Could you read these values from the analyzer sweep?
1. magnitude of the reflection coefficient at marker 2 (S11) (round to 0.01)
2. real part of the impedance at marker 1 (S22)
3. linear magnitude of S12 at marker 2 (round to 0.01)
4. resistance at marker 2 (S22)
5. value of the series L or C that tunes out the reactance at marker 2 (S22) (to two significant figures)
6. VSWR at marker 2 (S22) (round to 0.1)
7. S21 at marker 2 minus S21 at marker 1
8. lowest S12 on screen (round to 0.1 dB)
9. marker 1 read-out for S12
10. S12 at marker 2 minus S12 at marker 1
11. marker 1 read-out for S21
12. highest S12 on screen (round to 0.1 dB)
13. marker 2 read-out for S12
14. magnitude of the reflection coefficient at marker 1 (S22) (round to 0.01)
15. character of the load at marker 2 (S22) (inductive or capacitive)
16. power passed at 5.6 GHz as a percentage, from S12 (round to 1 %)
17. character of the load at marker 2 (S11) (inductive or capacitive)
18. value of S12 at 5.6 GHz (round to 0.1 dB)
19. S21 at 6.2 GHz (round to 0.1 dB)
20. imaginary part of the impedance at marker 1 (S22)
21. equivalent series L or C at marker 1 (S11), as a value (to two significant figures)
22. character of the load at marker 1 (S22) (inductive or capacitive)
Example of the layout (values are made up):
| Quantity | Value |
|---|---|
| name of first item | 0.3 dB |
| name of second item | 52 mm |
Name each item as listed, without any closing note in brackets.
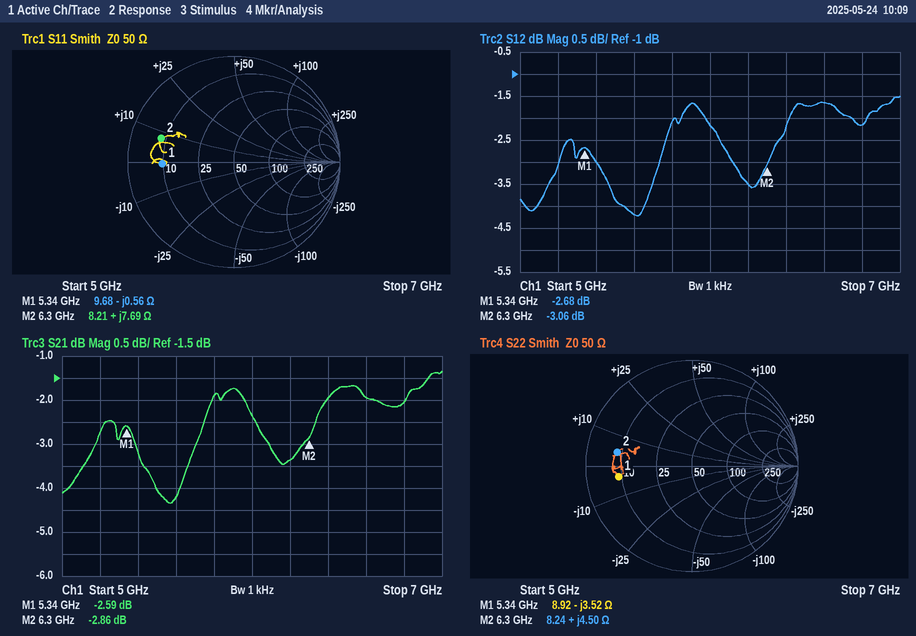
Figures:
| Quantity | Value |
|---|---|
| magnitude of the reflection coefficient at marker 2 (S11) | 0.72 |
| real part of the impedance at marker 1 | 8.92 Ω |
| linear magnitude of S12 at marker 2 | 0.70 |
| resistance at marker 2 | 8.24 Ω |
| value of the series L or C that tunes out the reactance at marker 2 (S22) | 5.6 pF |
| VSWR at marker 2 (S22) | 6.1 |
| S21 at marker 2 minus S21 at marker 1 | -0.27 dB |
| lowest S12 on screen | -4.2 dB |
| marker 1 read-out for S12 | -2.68 dB |
| S12 at marker 2 minus S12 at marker 1 | -0.38 dB |
| marker 1 read-out for S21 | -2.59 dB |
| highest S12 on screen | -1.5 dB |
| marker 2 read-out for S12 | -3.06 dB |
| magnitude of the reflection coefficient at marker 1 (S22) | 0.70 |
| character of the load at marker 2 (S22) | inductive |
| power passed at 5.6 GHz as a percentage, from S12 | 38 % |
| character of the load at marker 2 (S11) | inductive |
| value of S12 at 5.6 GHz | -4.2 dB |
| S21 at 6.2 GHz | -3.4 dB |
| imaginary part of the impedance at marker 1 | -3.52 Ω |
| equivalent series L or C at marker 1 (S11), as a value | 53 pF |
| character of the load at marker 1 (S22) | capacitive |
